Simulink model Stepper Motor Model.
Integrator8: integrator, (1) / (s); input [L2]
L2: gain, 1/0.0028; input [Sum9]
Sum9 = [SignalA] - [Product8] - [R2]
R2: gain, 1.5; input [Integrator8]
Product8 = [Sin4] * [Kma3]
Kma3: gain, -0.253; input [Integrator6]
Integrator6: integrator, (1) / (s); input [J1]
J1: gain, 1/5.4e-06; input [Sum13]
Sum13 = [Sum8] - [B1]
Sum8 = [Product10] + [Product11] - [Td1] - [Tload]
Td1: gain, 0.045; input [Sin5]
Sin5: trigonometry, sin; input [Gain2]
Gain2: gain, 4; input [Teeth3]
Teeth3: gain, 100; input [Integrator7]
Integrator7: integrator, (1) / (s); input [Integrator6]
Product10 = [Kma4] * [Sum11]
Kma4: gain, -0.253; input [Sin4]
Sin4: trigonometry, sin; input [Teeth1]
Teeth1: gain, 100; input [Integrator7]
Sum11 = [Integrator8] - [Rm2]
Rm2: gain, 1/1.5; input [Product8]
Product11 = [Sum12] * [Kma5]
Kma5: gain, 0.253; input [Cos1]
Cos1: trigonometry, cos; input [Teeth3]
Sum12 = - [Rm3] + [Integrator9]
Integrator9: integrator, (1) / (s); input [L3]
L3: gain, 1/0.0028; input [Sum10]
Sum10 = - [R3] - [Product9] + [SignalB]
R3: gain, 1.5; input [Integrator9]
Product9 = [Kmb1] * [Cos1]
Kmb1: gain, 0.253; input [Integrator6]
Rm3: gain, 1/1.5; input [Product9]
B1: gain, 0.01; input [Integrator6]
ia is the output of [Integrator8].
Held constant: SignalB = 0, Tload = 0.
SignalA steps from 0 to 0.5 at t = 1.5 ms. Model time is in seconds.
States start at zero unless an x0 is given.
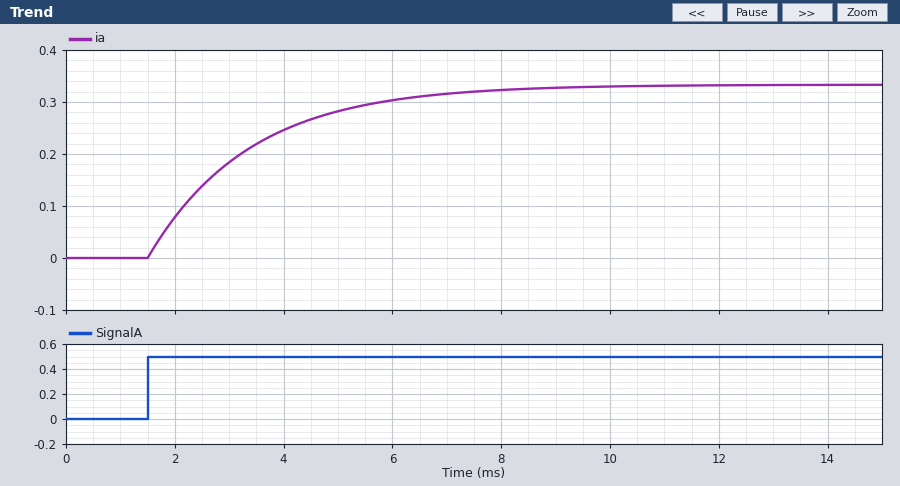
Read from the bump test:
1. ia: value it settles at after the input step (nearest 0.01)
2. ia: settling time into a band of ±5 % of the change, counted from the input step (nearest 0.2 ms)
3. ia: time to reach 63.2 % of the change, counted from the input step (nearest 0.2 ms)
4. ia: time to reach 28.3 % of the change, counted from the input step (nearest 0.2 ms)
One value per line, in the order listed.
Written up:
0.33
5.6 ms
1.8 ms
0.6 ms
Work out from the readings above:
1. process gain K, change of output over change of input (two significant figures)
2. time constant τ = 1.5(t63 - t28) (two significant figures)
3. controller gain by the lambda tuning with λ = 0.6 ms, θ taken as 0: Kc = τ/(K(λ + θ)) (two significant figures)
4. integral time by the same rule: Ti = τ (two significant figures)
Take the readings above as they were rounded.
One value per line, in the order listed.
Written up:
0.66
1.8 ms
4.5
1.8 ms
